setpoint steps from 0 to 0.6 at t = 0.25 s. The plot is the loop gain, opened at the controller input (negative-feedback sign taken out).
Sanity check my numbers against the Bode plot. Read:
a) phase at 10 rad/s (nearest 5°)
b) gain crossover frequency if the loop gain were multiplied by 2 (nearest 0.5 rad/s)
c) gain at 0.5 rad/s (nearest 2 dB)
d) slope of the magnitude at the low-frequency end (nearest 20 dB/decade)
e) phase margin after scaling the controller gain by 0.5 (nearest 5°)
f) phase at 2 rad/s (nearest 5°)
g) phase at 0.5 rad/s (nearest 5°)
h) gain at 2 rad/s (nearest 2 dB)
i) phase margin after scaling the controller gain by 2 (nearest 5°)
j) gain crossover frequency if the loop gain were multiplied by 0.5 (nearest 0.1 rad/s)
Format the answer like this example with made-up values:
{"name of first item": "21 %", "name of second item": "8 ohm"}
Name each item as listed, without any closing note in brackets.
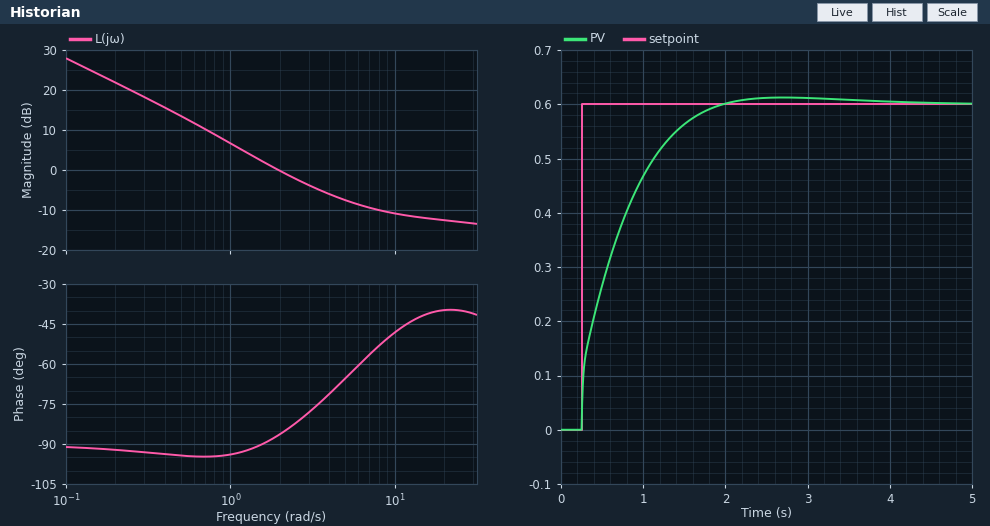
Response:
{"phase at 10 rad/s": "-50°", "gain crossover frequency if the loop gain were multiplied by 2": "4.0 rad/s", "gain at 0.5 rad/s": "14 dB", "slope of the magnitude at the low-frequency end": "-20 dB/decade", "phase margin after scaling the controller gain by 0.5": "85°", "phase at 2 rad/s": "-85°", "phase at 0.5 rad/s": "-95°", "gain at 2 rad/s": "0 dB", "phase margin after scaling the controller gain by 2": "110°", "gain crossover frequency if the loop gain were multiplied by 0.5": "1.1 rad/s"}
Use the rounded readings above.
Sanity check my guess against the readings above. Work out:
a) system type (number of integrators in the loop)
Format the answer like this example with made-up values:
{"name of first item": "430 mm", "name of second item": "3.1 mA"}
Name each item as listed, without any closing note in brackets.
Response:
{"system type": "1"}
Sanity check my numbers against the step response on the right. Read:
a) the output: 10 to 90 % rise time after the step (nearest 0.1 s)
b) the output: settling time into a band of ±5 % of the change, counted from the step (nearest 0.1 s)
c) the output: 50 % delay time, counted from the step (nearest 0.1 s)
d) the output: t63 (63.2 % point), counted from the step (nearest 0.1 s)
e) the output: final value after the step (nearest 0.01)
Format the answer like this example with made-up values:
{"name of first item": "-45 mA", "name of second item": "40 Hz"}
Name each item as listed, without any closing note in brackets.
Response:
{"the output: 10 to 90 % rise time after the step": "1.1 s", "the output: settling time into a band of ±5 % of the change, counted from the step": "1.3 s", "the output: 50 % delay time, counted from the step": "0.3 s", "the output: t63 (63.2 % point), counted from the step": "0.5 s", "the output: final value after the step": "0.60"}
